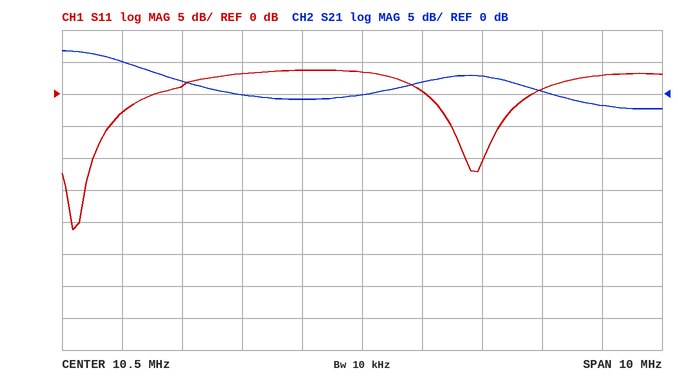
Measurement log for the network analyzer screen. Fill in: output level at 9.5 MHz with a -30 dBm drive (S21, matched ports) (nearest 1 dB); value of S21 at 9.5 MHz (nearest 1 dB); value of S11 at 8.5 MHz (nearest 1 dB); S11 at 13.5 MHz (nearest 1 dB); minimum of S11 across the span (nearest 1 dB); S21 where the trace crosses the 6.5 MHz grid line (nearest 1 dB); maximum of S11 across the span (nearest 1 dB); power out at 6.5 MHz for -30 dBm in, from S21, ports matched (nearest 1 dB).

-31 dBm
-1 dB
3 dB
1 dB
-21 dB
5 dB
4 dB
-25 dBm
